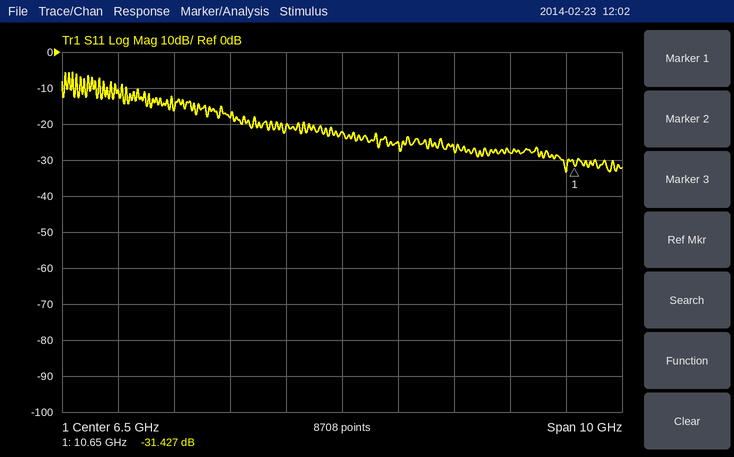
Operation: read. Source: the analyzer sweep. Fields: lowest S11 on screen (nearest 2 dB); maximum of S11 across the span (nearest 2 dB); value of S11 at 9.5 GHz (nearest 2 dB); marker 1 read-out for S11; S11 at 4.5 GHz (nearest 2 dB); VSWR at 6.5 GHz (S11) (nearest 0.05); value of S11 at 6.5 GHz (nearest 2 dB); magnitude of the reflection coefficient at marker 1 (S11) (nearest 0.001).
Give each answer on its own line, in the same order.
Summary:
-34 dB
-6 dB
-28 dB
-31.427 dB
-18 dB
1.15
-22 dB
0.027
